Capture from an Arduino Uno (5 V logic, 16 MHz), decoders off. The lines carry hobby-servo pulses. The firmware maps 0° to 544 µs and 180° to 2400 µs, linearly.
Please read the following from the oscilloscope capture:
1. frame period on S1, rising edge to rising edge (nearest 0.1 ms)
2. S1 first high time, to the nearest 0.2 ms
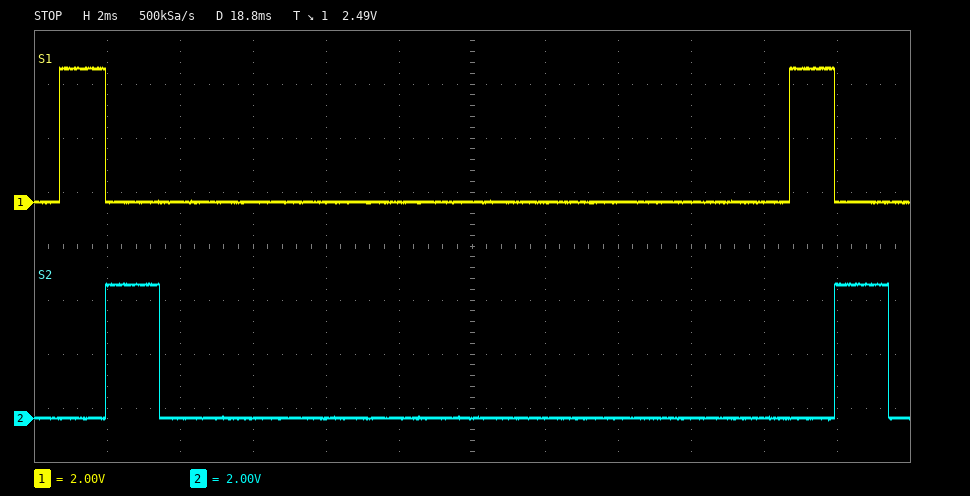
20.0 ms
1.2 ms
